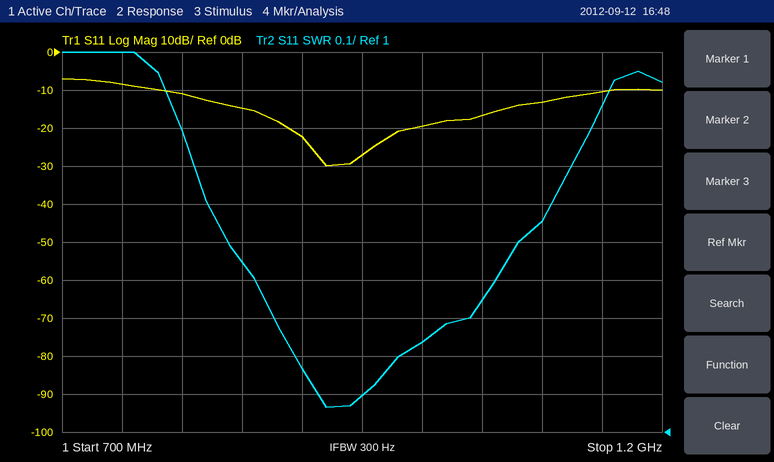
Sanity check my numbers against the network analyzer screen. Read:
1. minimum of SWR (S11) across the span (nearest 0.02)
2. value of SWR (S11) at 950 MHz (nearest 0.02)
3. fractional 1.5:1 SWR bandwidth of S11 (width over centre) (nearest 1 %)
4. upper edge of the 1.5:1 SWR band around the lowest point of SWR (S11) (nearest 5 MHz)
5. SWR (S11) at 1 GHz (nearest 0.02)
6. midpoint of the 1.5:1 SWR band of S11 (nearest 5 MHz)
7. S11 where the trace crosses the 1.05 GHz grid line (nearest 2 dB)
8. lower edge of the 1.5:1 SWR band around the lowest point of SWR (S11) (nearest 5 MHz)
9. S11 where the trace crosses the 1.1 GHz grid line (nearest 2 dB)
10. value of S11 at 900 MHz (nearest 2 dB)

1.06
1.10
25 %
1.080 GHz
1.24
960 MHz
-16 dB
840 MHz
-14 dB
-22 dB
